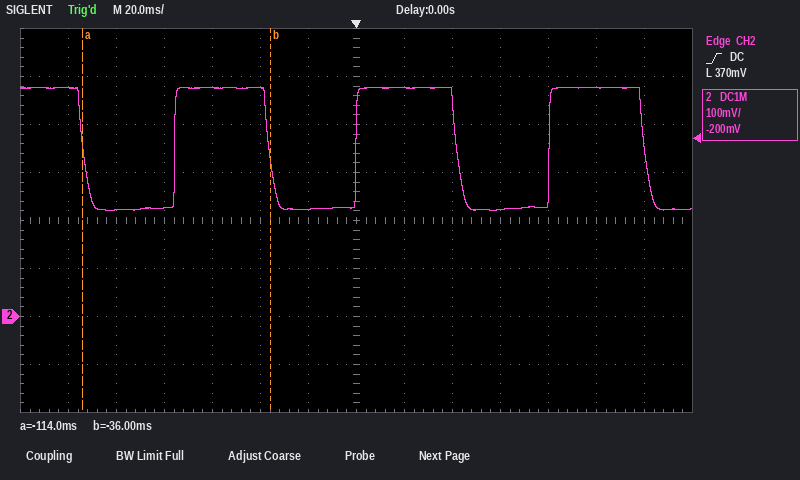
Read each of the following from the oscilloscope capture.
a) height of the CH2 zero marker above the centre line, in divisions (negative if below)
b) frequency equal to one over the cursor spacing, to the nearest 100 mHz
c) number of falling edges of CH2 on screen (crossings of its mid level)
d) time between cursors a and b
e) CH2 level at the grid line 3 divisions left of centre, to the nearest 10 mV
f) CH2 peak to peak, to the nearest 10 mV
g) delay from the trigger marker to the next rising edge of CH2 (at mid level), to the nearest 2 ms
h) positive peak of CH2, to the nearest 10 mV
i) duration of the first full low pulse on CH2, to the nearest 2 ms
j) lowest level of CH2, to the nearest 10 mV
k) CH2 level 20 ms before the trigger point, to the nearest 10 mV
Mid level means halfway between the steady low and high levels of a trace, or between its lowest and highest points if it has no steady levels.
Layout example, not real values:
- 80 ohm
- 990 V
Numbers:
- -2.0 div
- 12.8 Hz
- 4
- 78 ms
- 480 mV
- 260 mV
- 80 ms
- 480 mV
- 38 ms
- 220 mV
- 220 mV
